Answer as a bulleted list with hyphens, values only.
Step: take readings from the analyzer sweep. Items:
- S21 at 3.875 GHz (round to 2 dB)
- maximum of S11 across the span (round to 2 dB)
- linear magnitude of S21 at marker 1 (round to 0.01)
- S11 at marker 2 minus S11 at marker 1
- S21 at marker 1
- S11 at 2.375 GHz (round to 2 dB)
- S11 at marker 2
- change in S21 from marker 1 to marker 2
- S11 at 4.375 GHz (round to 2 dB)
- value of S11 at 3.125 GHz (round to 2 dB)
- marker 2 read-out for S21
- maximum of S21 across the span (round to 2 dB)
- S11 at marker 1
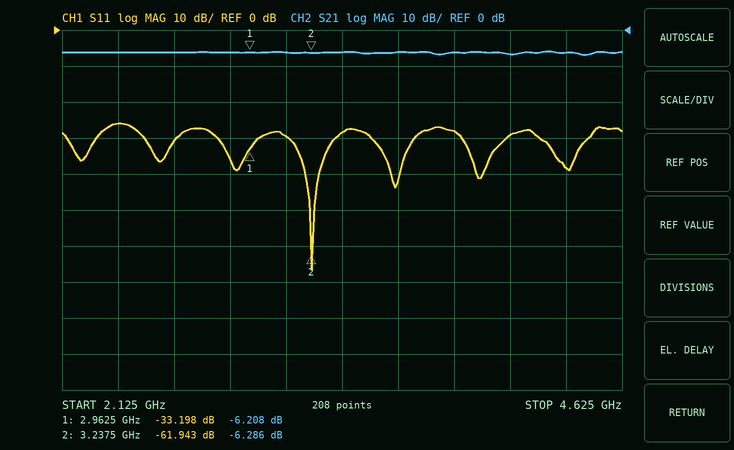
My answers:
- -6 dB
- -26 dB
- 0.49
- -28.745 dB
- -6.208 dB
- -26 dB
- -61.943 dB
- -0.078 dB
- -38 dB
- -30 dB
- -6.286 dB
- -6 dB
- -33.198 dB
